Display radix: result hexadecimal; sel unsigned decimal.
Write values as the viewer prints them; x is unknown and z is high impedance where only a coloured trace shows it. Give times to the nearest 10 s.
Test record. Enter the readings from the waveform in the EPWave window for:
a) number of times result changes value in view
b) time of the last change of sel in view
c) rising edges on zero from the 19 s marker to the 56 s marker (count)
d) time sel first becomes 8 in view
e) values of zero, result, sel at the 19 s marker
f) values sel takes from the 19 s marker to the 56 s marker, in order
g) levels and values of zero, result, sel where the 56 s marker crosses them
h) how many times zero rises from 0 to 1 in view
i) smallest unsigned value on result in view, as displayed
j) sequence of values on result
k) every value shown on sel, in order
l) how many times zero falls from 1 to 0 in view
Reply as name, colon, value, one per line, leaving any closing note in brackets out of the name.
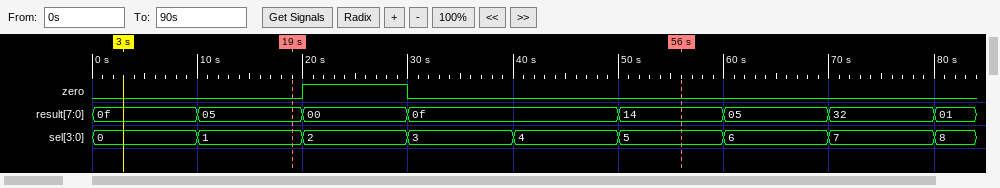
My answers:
number of times result changes value in view: 7
time of the last change of sel in view: 80 s
rising edges on zero from the 19 s marker to the 56 s marker: 1
time sel first becomes 8 in view: 80 s
values of zero, result, sel at the 19 s marker: zero=0, result=05, sel=1
values sel takes from the 19 s marker to the 56 s marker, in order: 1, 2, 3, 4, 5
levels and values of zero, result, sel where the 56 s marker crosses them: zero=0, result=14, sel=5
how many times zero rises from 0 to 1 in view: 1
smallest unsigned value on result in view, as displayed: 00
sequence of values on result: 0f, 05, 00, 0f, 14, 05, 32, 01
every value shown on sel, in order: 0, 1, 2, 3, 4, 5, 6, 7, 8
how many times zero falls from 1 to 0 in view: 1
